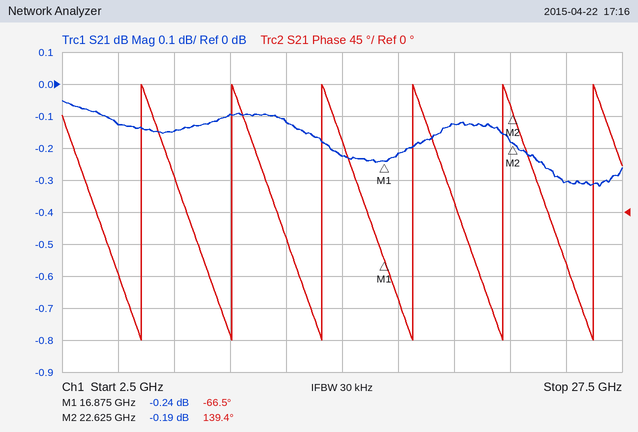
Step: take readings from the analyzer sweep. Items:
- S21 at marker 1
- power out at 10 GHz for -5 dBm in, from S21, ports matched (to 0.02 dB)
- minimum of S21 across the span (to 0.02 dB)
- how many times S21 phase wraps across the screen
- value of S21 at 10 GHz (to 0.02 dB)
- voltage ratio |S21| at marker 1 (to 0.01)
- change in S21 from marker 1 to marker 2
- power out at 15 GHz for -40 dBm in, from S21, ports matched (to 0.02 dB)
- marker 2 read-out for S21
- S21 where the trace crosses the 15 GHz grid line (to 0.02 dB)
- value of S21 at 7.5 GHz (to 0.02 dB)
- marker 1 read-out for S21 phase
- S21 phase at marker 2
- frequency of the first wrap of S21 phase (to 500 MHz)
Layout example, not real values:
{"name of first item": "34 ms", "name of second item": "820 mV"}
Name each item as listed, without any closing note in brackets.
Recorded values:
{"S21 at marker 1": "-0.24 dB", "power out at 10 GHz for -5 dBm in, from S21, ports matched": "-5.10 dBm", "minimum of S21 across the span": "-0.32 dB", "how many times S21 phase wraps across the screen": "6", "value of S21 at 10 GHz": "-0.10 dB", "voltage ratio |S21| at marker 1": "0.97", "change in S21 from marker 1 to marker 2": "0.05 dB", "power out at 15 GHz for -40 dBm in, from S21, ports matched": "-40.22 dBm", "marker 2 read-out for S21": "-0.19 dB", "S21 where the trace crosses the 15 GHz grid line": "-0.22 dB", "value of S21 at 7.5 GHz": "-0.14 dB", "marker 1 read-out for S21 phase": "-66.5°", "S21 phase at marker 2": "139.4°", "frequency of the first wrap of S21 phase": "6.0 GHz"}
